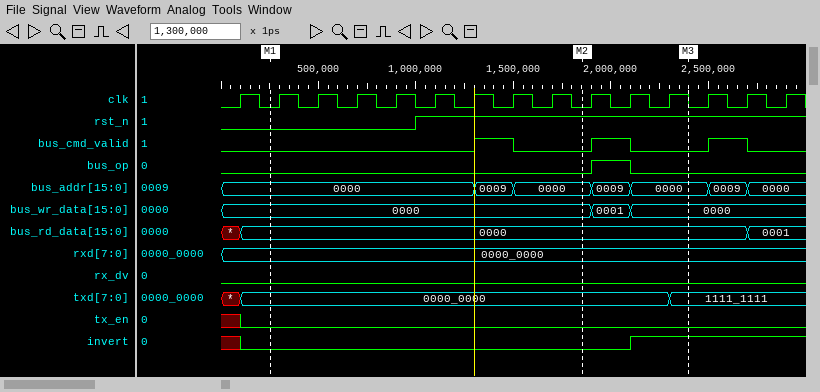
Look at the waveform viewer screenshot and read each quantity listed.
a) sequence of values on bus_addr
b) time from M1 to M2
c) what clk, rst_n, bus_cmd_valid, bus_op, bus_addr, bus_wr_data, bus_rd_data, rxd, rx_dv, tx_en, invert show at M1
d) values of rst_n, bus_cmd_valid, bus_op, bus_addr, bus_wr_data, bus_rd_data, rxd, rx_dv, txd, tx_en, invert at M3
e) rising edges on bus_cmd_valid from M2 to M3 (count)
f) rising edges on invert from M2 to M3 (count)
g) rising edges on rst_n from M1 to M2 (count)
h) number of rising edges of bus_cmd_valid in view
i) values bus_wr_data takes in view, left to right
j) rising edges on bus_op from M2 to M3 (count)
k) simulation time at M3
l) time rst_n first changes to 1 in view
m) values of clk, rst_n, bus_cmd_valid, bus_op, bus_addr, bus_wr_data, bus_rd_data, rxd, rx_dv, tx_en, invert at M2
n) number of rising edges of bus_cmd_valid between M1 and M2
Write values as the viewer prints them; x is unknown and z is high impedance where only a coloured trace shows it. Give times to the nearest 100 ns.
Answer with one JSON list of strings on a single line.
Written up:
["0000, 0009, 0000, 0009, 0000, 0009, 0000", "1600 ns", "clk=0, rst_n=0, bus_cmd_valid=0, bus_op=0, bus_addr=0000, bus_wr_data=0000, bus_rd_data=0000, rxd=0000_0000, rx_dv=0, tx_en=0, invert=0", "rst_n=1, bus_cmd_valid=0, bus_op=0, bus_addr=0000, bus_wr_data=0000, bus_rd_data=0000, rxd=0000_0000, rx_dv=0, txd=1111_1111, tx_en=0, invert=1", "1", "1", "1", "3", "0000, 0001, 0000", "1", "2400 ns", "1000 ns", "clk=0, rst_n=1, bus_cmd_valid=0, bus_op=0, bus_addr=0000, bus_wr_data=0000, bus_rd_data=0000, rxd=0000_0000, rx_dv=0, tx_en=0, invert=0", "1"]
